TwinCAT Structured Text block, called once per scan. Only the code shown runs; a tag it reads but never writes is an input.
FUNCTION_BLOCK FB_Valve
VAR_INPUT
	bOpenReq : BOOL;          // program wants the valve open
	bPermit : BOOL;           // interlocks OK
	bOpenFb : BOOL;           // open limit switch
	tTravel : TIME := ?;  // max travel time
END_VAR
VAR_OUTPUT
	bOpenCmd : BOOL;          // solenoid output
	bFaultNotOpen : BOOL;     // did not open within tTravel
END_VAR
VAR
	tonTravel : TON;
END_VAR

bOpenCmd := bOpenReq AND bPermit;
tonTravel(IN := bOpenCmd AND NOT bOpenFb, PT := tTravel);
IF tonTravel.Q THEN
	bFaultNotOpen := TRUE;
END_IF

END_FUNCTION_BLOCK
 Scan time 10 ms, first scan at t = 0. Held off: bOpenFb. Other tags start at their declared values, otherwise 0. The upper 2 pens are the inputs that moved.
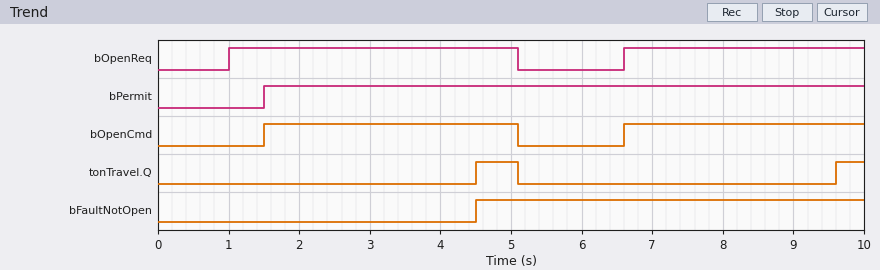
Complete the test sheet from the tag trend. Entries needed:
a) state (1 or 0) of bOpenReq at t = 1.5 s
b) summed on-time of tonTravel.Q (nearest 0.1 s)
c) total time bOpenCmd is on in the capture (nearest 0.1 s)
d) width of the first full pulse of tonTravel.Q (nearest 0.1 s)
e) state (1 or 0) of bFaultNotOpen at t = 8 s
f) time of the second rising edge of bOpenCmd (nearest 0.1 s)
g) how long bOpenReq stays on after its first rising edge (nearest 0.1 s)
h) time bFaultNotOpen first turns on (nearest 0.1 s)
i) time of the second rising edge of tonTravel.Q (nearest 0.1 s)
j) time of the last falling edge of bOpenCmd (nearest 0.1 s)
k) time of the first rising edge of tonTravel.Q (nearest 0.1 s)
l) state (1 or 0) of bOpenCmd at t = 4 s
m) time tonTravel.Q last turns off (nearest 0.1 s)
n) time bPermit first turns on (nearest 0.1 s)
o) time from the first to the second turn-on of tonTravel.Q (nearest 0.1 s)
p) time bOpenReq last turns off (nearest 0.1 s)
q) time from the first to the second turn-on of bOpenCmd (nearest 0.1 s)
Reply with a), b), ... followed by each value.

a) 1
b) 1.0 s
c) 7.0 s
d) 0.6 s
e) 1
f) 6.6 s
g) 4.1 s
h) 4.5 s
i) 9.6 s
j) 5.1 s
k) 4.5 s
l) 1
m) 5.1 s
n) 1.5 s
o) 5.1 s
p) 5.1 s
q) 5.1 s
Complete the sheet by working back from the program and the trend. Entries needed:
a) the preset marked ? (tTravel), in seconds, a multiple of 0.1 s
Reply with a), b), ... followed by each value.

a) 3.0 s
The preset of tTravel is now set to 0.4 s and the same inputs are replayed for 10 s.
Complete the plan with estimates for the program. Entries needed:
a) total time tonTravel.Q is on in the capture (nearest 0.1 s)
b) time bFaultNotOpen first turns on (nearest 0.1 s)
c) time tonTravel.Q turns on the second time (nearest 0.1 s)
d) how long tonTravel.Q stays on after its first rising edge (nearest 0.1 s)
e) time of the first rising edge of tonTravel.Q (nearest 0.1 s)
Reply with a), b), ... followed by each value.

a) 6.2 s
b) 1.9 s
c) 7.0 s
d) 3.2 s
e) 1.9 s
